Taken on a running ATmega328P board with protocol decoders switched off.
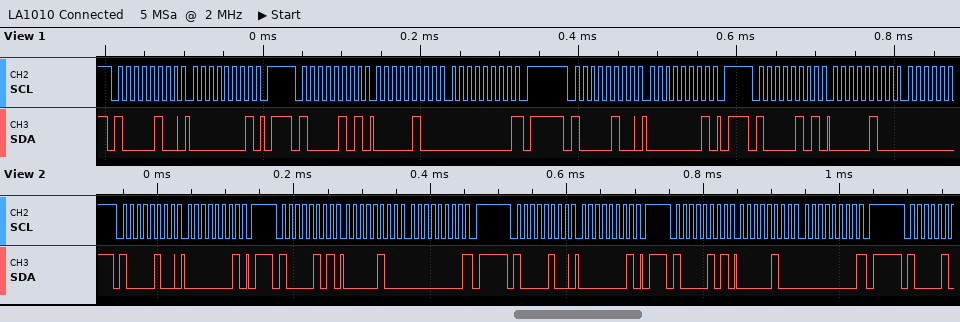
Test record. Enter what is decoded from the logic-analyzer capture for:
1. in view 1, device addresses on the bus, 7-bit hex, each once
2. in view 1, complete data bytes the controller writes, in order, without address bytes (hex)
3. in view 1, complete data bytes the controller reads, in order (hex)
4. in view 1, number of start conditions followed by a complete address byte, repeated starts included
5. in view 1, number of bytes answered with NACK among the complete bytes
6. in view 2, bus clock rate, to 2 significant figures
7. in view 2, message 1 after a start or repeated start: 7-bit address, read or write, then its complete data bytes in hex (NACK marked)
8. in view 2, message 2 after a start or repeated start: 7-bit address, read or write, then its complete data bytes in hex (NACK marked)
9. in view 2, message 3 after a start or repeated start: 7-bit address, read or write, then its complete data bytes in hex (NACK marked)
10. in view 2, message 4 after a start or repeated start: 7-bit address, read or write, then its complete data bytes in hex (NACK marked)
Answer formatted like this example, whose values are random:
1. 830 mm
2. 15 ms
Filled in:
1. 0x42
2. 01 01
3. 04 00 04
4. 4
5. 1
6. 100 kHz
7. 0x42 write: 01
8. 0x42 read: 04 00 NACK
9. 0x42 write: 01
10. 0x42 read: 04 00 NACK
